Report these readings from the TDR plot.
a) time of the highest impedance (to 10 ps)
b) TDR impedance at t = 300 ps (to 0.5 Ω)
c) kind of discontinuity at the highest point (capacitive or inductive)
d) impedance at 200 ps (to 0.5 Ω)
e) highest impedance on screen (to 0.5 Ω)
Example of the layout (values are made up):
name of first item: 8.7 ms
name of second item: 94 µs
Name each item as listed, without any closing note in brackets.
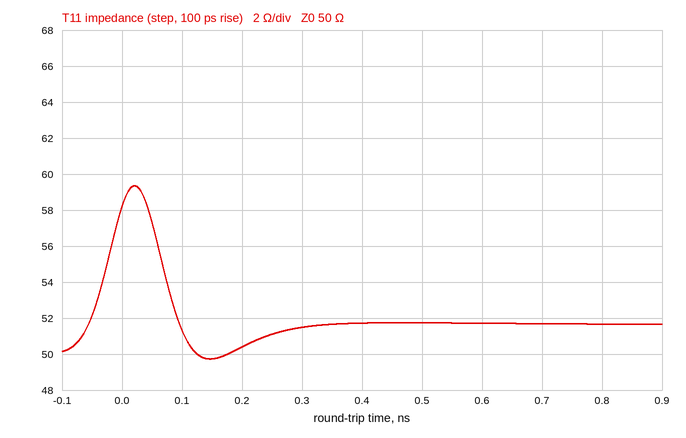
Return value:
time of the highest impedance: 20 ps
TDR impedance at t = 300 ps: 51.5 Ω
kind of discontinuity at the highest point: inductive
impedance at 200 ps: 50.5 Ω
highest impedance on screen: 59.5 Ω
